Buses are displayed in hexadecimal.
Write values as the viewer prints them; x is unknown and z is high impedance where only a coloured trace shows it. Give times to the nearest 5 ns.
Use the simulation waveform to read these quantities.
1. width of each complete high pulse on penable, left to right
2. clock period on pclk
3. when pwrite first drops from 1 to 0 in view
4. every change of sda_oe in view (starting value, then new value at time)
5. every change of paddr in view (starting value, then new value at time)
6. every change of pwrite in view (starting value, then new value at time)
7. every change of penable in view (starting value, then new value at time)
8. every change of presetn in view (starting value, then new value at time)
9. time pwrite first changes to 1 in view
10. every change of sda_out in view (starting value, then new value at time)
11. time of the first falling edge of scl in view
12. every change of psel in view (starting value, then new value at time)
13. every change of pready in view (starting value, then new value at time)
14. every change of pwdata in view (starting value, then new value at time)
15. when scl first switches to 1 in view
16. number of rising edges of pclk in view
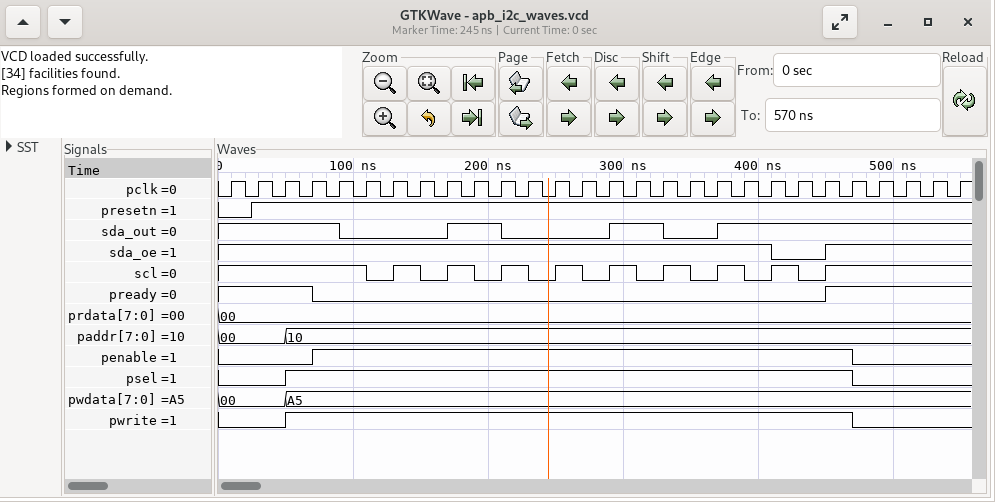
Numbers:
400 ns
20 ns
470 ns
1, 0 at 410 ns, 1 at 450 ns
00, 10 at 50 ns
0, 1 at 50 ns, 0 at 470 ns
0, 1 at 70 ns, 0 at 470 ns
0, 1 at 25 ns
50 ns
1, 0 at 90 ns, 1 at 170 ns, 0 at 210 ns, 1 at 290 ns, 0 at 330 ns, 1 at 370 ns
110 ns
0, 1 at 50 ns, 0 at 470 ns
1, 0 at 70 ns, 1 at 450 ns
00, A5 at 50 ns
130 ns
28
